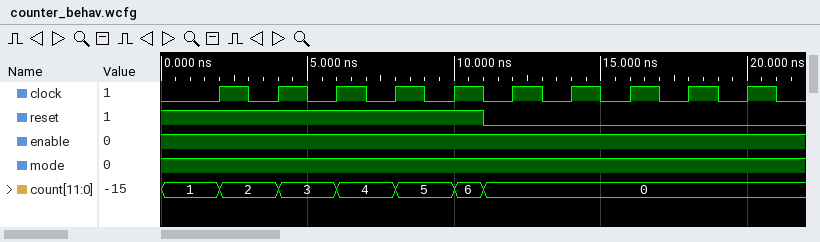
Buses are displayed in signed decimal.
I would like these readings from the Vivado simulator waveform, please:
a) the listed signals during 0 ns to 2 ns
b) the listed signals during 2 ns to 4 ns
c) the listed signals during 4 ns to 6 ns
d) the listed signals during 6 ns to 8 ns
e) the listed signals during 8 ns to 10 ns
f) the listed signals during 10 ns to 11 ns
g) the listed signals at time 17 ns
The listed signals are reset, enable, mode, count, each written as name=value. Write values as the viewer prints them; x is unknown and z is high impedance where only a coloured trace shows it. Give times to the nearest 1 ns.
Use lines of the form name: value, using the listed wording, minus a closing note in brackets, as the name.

the listed signals during 0 ns to 2 ns: reset=1, enable=1, mode=1, count=1
the listed signals during 2 ns to 4 ns: reset=1, enable=1, mode=1, count=2
the listed signals during 4 ns to 6 ns: reset=1, enable=1, mode=1, count=3
the listed signals during 6 ns to 8 ns: reset=1, enable=1, mode=1, count=4
the listed signals during 8 ns to 10 ns: reset=1, enable=1, mode=1, count=5
the listed signals during 10 ns to 11 ns: reset=1, enable=1, mode=1, count=6
the listed signals at time 17 ns: reset=0, enable=1, mode=1, count=0
